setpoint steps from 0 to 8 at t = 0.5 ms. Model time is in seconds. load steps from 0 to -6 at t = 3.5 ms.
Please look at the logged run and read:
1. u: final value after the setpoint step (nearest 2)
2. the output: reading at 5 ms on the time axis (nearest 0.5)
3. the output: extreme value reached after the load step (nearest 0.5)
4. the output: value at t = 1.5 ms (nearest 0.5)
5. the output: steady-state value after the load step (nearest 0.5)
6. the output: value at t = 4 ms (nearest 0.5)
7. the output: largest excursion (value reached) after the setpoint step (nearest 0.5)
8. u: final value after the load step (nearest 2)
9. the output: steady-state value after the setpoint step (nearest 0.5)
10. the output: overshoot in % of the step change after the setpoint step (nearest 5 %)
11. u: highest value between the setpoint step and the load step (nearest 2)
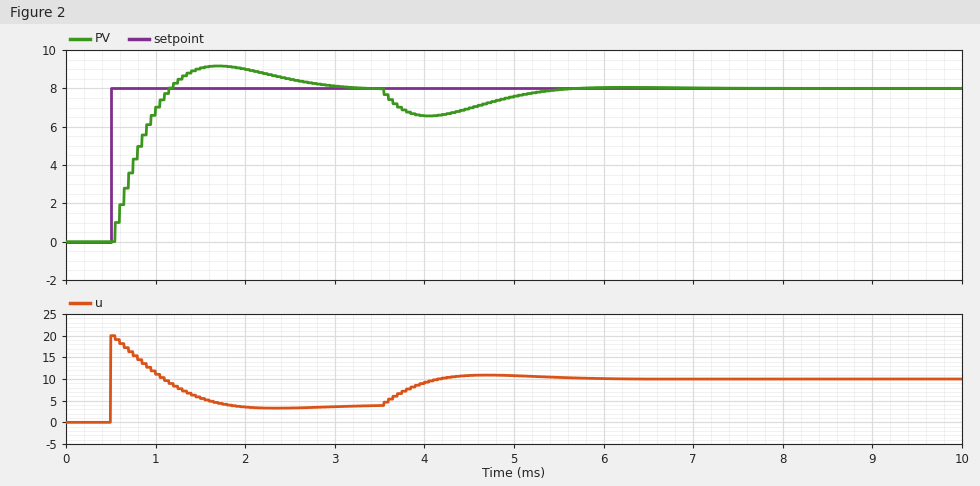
4
7.5
6.5
9.0
8.0
6.5
9.0
10
8.0
15 %
20
